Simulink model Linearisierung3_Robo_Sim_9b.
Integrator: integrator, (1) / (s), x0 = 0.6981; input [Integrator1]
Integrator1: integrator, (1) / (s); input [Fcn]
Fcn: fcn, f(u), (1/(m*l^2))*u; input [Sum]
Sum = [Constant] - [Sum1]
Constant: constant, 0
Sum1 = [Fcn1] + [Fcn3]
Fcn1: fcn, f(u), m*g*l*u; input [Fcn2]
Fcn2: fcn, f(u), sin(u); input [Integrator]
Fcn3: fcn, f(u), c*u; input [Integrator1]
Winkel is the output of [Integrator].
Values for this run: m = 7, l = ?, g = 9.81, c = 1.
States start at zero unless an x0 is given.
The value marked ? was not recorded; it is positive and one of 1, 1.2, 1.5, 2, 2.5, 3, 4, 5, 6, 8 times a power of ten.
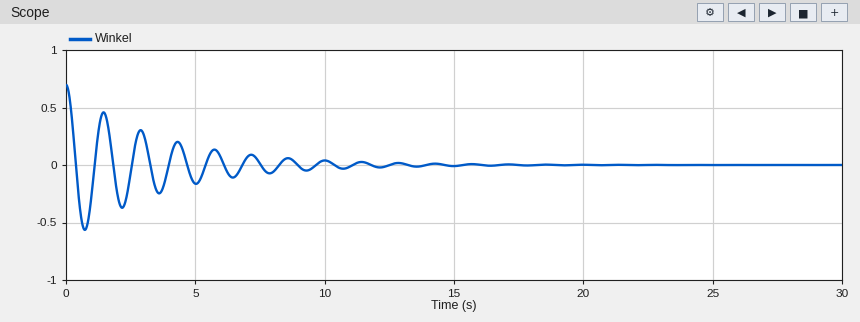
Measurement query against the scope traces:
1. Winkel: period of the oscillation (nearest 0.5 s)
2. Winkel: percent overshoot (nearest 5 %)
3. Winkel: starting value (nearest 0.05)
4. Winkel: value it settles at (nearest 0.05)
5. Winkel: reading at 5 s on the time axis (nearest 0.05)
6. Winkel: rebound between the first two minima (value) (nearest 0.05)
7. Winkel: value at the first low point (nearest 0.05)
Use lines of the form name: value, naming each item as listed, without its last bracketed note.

Winkel: period of the oscillation: 1.5 s
Winkel: percent overshoot: 80 %
Winkel: starting value: 0.70
Winkel: value it settles at: 0.00
Winkel: reading at 5 s on the time axis: -0.15
Winkel: rebound between the first two minima (value): 0.45
Winkel: value at the first low point: -0.55
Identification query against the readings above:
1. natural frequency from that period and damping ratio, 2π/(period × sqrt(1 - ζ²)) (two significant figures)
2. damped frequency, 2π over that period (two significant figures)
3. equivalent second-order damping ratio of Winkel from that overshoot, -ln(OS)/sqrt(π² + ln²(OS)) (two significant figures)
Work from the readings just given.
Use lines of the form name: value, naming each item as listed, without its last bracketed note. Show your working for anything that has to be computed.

natural frequency from that period and damping ratio, 2π/(period × sqrt(1 - ζ²)): 2π / (1.5 × sqrt(1 - 0.071²)) = 4.2 rad/s
damped frequency, 2π over that period: 2π / 1.5 = 4.2 rad/s
equivalent second-order damping ratio of Winkel from that overshoot, -ln(OS)/sqrt(π² + ln²(OS)): ln(0.8) = -0.223; 0.223 / sqrt(9.870 + 0.050) = 0.071
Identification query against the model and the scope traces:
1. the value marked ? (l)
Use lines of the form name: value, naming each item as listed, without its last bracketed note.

the value marked ?: 0.5
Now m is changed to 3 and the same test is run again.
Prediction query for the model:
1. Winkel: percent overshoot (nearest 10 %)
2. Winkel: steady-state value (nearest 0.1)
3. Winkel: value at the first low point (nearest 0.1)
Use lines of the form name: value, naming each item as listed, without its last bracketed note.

Winkel: percent overshoot: 60 %
Winkel: steady-state value: 0.0
Winkel: value at the first low point: -0.4
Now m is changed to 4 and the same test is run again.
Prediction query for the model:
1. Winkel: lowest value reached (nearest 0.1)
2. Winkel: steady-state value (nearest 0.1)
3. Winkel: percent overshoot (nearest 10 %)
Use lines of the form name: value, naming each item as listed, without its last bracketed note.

Winkel: lowest value reached: -0.5
Winkel: steady-state value: 0.0
Winkel: percent overshoot: 70 %
